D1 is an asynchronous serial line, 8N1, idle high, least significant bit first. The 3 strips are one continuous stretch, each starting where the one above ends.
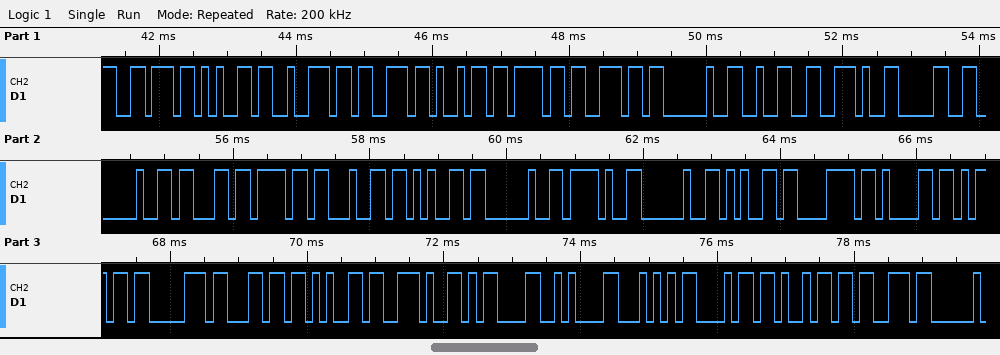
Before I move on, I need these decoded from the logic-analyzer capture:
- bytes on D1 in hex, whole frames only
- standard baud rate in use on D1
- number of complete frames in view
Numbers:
76 65 72 73 69 6F 6E 20 32 2E 30 20 63 6F 64 65 20 2F 20 65 78 61 6D 70 6C 65 2E 0D 0A 54 68 69 73
9600 baud
33
